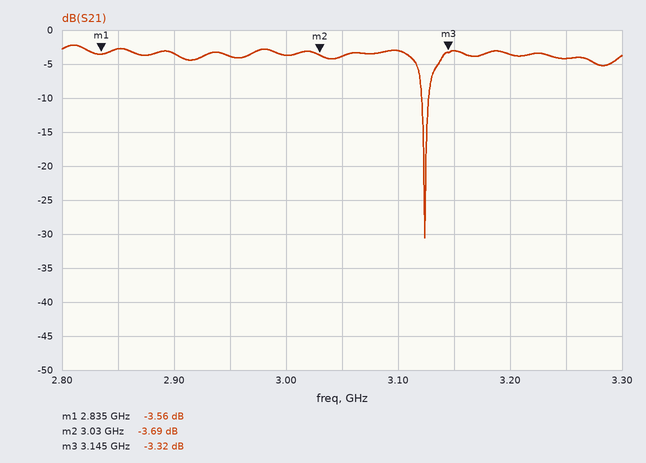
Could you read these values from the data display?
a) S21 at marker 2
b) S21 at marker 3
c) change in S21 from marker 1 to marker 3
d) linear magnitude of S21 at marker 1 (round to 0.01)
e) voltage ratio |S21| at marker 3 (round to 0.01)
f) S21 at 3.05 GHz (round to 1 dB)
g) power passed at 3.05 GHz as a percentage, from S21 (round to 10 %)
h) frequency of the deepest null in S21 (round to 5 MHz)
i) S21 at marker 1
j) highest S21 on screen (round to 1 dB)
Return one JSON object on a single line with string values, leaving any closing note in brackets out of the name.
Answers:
{"S21 at marker 2": "-3.69 dB", "S21 at marker 3": "-3.32 dB", "change in S21 from marker 1 to marker 3": "0.24 dB", "linear magnitude of S21 at marker 1": "0.66", "voltage ratio |S21| at marker 3": "0.68", "S21 at 3.05 GHz": "-4 dB", "power passed at 3.05 GHz as a percentage, from S21": "40 %", "frequency of the deepest null in S21": "3.125 GHz", "S21 at marker 1": "-3.56 dB", "highest S21 on screen": "-2 dB"}
